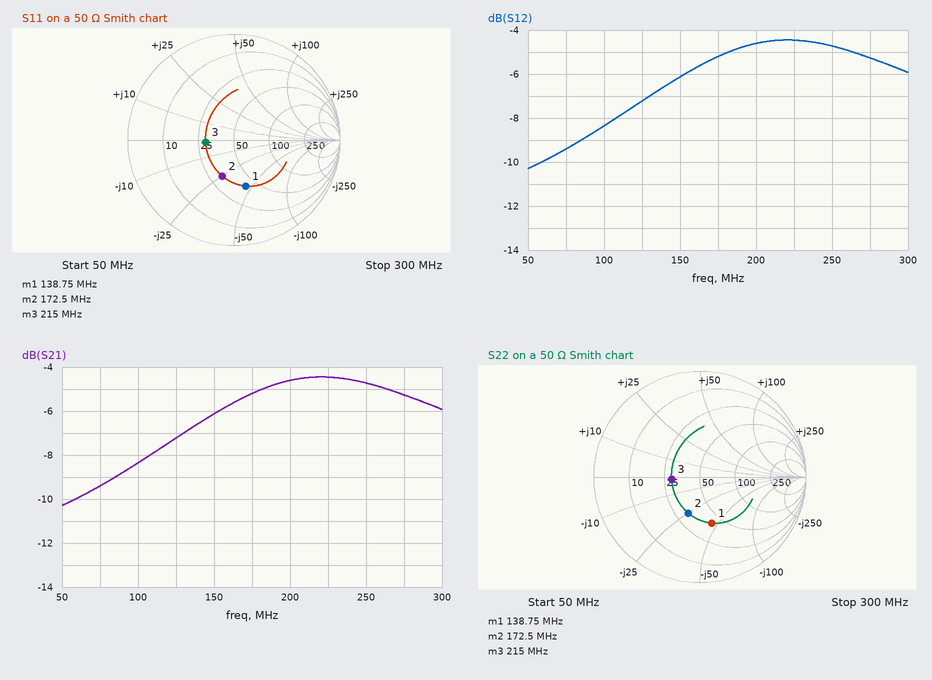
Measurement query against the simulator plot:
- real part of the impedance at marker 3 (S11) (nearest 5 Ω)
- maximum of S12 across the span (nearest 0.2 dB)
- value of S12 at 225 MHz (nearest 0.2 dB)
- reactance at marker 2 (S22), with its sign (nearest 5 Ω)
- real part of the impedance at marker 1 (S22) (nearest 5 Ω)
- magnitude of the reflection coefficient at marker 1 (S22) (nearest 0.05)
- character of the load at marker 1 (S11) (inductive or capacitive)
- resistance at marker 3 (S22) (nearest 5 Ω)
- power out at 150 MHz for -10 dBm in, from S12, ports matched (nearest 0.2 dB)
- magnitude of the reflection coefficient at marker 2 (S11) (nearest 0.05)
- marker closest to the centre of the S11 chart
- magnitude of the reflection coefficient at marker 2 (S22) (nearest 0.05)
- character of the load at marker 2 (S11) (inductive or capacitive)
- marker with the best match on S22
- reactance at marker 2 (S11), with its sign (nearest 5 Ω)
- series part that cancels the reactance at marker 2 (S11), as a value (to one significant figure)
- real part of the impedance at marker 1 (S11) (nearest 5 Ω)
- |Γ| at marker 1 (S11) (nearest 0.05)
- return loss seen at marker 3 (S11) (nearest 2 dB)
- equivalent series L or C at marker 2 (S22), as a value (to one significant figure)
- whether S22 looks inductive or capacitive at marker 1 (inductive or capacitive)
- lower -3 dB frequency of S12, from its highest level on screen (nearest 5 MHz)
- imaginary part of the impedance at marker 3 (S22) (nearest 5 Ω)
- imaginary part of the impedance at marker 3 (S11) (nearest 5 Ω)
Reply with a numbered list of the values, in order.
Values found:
1. 30 Ω
2. -4.4 dB
3. -4.4 dB
4. -25 Ω
5. 40 Ω
6. 0.45
7. capacitive
8. 30 Ω
9. -16.2 dBm
10. 0.35
11. marker 3
12. 0.35
13. capacitive
14. marker 3
15. -25 Ω
16. 20 nH
17. 40 Ω
18. 0.45
19. 12 dB
20. 40 pF
21. capacitive
22. 120 MHz
23. 0 Ω
24. 0 Ω
